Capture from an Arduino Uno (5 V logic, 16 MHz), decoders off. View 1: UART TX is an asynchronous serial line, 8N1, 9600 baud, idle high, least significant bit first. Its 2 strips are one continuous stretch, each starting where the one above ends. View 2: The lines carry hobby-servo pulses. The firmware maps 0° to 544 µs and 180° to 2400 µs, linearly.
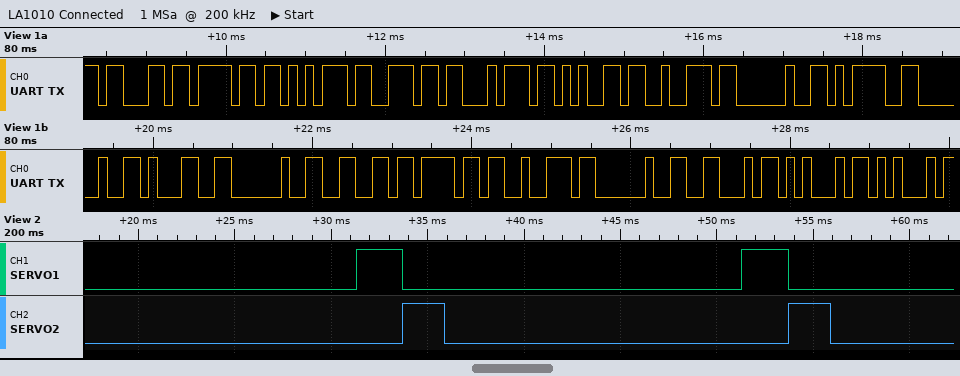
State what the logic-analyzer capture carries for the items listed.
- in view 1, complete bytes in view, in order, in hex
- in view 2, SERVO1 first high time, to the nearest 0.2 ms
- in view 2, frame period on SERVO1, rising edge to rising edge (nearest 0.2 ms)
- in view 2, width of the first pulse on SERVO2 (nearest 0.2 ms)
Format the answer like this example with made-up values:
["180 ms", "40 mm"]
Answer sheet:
["63 6F 75 6E 74 65 72 20 3D 20 31 20 66 6F 72 20 46 45 45", "2.4 ms", "20.0 ms", "2.2 ms"]
